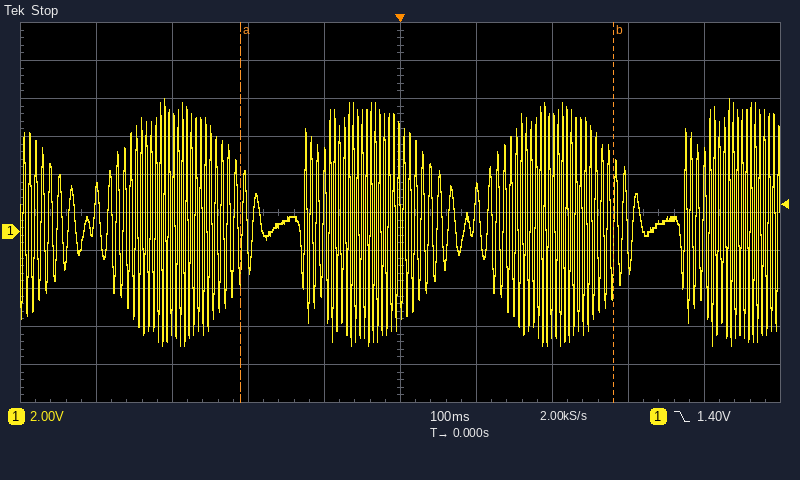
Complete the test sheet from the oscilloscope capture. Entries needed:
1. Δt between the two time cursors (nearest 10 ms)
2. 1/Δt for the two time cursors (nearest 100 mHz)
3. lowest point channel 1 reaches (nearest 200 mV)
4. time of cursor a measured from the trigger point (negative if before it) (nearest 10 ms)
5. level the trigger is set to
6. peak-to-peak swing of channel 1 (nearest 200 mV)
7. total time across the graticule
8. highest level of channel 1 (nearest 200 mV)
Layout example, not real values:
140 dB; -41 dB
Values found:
490 ms; 2.0 Hz; -6.0 V; -210 ms; 1.40 V; 13.0 V; 1 s; 7.0 V
